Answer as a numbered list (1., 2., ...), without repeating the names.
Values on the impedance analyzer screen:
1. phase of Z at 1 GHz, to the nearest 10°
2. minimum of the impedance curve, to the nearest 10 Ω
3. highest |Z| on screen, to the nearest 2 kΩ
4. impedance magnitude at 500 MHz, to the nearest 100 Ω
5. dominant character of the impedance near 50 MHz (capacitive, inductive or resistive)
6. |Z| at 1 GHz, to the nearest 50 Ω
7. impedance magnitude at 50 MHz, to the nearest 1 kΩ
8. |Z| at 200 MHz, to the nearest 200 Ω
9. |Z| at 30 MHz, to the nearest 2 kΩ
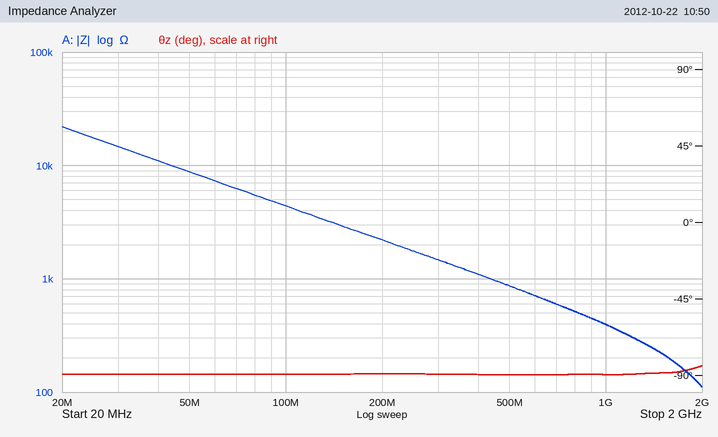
1. -90°
2. 110 Ω
3. 22 kΩ
4. 900 Ω
5. capacitive
6. 400 Ω
7. 9 kΩ
8. 2.2 kΩ
9. 14 kΩ
